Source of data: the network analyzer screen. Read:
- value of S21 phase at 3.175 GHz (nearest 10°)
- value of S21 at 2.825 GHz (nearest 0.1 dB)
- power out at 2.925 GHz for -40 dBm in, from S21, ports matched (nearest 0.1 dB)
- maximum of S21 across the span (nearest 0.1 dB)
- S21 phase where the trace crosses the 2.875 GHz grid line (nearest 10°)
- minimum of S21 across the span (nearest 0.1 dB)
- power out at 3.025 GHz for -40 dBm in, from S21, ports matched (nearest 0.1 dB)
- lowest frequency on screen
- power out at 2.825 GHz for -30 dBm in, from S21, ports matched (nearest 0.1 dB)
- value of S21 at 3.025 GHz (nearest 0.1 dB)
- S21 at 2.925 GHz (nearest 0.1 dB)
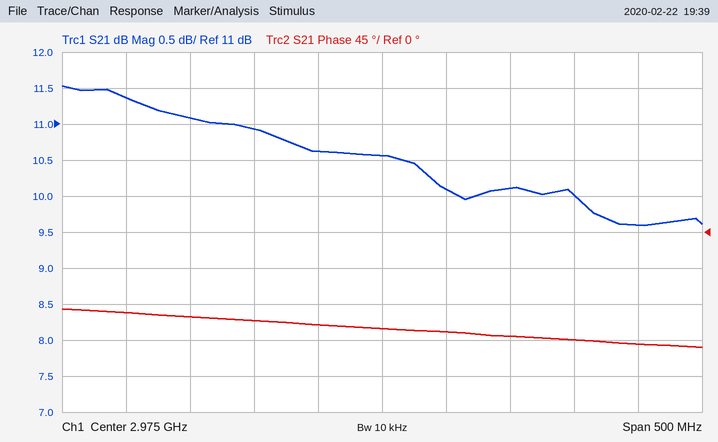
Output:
-140°
11.1 dB
-29.4 dBm
11.5 dB
-110°
9.6 dB
-29.9 dBm
2.725 GHz
-18.9 dBm
10.1 dB
10.6 dB
